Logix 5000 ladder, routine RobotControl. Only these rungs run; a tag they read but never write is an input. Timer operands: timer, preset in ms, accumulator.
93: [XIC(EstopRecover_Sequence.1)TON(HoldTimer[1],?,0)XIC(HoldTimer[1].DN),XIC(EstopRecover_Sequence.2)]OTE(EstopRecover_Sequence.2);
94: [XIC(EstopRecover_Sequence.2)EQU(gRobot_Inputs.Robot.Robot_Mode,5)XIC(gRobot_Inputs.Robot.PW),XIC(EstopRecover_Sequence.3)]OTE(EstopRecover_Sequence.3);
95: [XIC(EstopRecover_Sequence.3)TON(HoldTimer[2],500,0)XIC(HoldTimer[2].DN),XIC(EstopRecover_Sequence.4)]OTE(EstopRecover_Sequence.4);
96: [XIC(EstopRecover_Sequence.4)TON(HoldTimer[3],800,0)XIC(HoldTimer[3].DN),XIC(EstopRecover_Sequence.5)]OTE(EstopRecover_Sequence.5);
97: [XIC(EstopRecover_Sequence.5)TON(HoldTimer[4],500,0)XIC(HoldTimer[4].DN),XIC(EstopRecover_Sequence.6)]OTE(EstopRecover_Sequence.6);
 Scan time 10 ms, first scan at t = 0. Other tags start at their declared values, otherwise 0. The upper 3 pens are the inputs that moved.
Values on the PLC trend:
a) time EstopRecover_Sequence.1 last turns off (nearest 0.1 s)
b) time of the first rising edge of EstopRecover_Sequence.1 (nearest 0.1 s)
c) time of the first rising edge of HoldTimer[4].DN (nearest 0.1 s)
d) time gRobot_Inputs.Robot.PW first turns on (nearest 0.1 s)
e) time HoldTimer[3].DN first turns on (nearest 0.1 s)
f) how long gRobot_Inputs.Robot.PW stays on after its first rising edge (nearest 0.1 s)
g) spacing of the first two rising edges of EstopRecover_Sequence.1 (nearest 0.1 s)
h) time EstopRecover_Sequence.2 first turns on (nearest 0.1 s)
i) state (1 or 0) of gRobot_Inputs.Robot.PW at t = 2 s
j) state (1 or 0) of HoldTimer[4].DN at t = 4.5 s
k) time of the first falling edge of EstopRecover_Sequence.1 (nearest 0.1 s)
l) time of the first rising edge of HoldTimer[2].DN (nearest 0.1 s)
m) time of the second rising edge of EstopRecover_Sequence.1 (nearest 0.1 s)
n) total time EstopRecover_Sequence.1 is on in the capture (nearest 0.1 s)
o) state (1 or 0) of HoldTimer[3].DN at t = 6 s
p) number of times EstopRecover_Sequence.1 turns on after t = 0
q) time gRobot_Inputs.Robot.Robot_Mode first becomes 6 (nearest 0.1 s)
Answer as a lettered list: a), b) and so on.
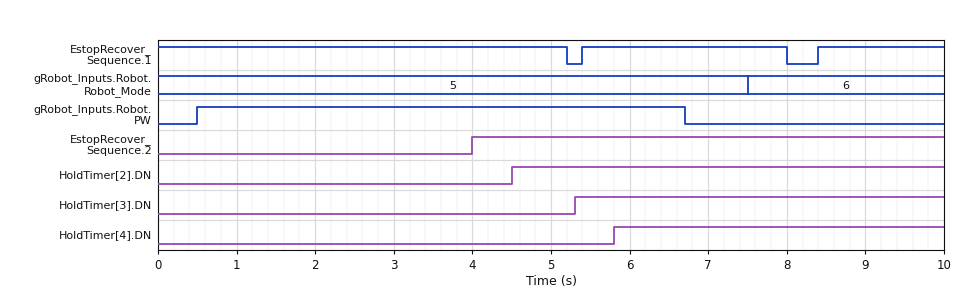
a) 8.0 s
b) 5.4 s
c) 5.8 s
d) 0.5 s
e) 5.3 s
f) 6.2 s
g) 3.0 s
h) 4.0 s
i) 1
j) 0
k) 5.2 s
l) 4.5 s
m) 8.4 s
n) 9.4 s
o) 1
p) 2
q) 7.5 s
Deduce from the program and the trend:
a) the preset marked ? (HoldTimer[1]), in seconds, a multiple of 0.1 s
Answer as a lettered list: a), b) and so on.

a) 4.0 s
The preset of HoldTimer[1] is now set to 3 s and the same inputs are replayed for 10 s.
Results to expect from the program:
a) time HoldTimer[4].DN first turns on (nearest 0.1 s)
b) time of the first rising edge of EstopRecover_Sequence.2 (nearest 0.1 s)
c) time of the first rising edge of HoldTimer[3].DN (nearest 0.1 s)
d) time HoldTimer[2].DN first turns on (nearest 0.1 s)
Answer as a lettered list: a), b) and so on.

a) 4.8 s
b) 3.0 s
c) 4.3 s
d) 3.5 s
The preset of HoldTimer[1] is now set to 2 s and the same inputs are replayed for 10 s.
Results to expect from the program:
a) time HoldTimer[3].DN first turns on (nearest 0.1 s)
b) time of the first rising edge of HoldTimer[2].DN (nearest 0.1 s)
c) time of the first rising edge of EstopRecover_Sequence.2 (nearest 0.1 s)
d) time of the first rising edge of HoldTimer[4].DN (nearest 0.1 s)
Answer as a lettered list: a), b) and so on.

a) 3.3 s
b) 2.5 s
c) 2.0 s
d) 3.8 s
